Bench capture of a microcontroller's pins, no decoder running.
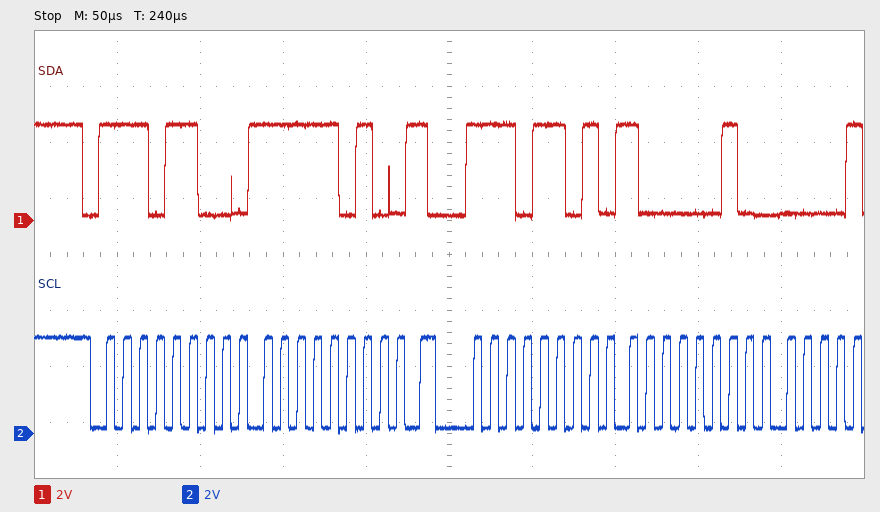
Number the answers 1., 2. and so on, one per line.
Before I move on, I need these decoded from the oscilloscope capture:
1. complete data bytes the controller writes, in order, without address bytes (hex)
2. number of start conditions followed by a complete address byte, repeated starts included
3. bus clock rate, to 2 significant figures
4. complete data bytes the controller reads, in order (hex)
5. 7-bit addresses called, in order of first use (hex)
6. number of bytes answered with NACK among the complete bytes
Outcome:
1. FA
2. 2
3. 100 kHz
4. 82
5. 0x76
6. 0
